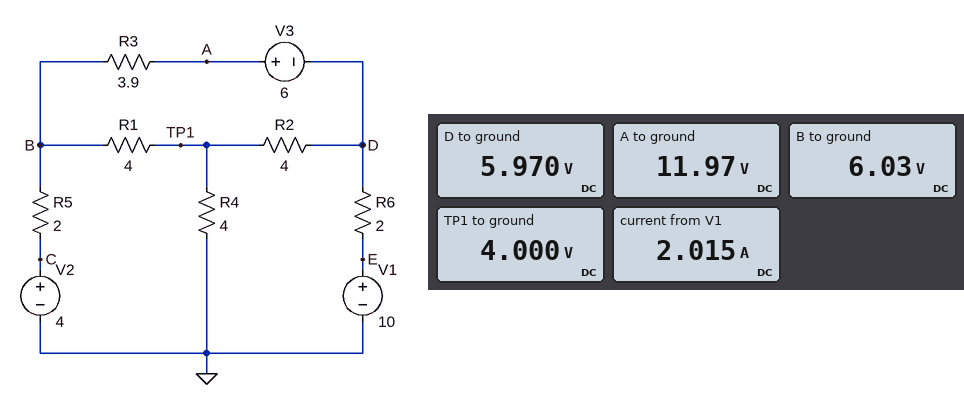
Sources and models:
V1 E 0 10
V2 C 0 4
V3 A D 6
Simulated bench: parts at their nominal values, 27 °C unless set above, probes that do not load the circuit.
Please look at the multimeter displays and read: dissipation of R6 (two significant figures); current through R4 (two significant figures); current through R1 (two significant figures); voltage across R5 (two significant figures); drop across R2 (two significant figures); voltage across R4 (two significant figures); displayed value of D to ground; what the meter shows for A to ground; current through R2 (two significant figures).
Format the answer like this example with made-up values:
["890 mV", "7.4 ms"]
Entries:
["8.1 W", "1.0 A", "510 mA", "2.0 V", "2.0 V", "4.0 V", "5.970 V", "11.97 V", "490 mA"]
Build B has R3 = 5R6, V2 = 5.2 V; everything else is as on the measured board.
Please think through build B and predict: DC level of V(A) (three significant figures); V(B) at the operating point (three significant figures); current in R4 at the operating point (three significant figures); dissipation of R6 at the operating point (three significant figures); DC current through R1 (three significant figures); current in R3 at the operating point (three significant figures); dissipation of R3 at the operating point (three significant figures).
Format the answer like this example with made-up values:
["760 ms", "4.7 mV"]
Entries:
["12.6 V", "6.40 V", "1.09 A", "5.68 W", "514 mA", "1.11 A", "6.94 W"]
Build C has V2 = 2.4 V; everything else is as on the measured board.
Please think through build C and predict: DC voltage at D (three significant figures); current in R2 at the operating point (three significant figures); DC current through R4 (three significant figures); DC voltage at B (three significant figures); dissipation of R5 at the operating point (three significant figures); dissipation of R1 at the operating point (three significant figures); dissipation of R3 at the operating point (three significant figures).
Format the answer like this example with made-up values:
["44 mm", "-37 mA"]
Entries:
["5.60 V", "514 mA", "886 mA", "5.03 V", "3.45 W", "551 mW", "11.1 W"]
